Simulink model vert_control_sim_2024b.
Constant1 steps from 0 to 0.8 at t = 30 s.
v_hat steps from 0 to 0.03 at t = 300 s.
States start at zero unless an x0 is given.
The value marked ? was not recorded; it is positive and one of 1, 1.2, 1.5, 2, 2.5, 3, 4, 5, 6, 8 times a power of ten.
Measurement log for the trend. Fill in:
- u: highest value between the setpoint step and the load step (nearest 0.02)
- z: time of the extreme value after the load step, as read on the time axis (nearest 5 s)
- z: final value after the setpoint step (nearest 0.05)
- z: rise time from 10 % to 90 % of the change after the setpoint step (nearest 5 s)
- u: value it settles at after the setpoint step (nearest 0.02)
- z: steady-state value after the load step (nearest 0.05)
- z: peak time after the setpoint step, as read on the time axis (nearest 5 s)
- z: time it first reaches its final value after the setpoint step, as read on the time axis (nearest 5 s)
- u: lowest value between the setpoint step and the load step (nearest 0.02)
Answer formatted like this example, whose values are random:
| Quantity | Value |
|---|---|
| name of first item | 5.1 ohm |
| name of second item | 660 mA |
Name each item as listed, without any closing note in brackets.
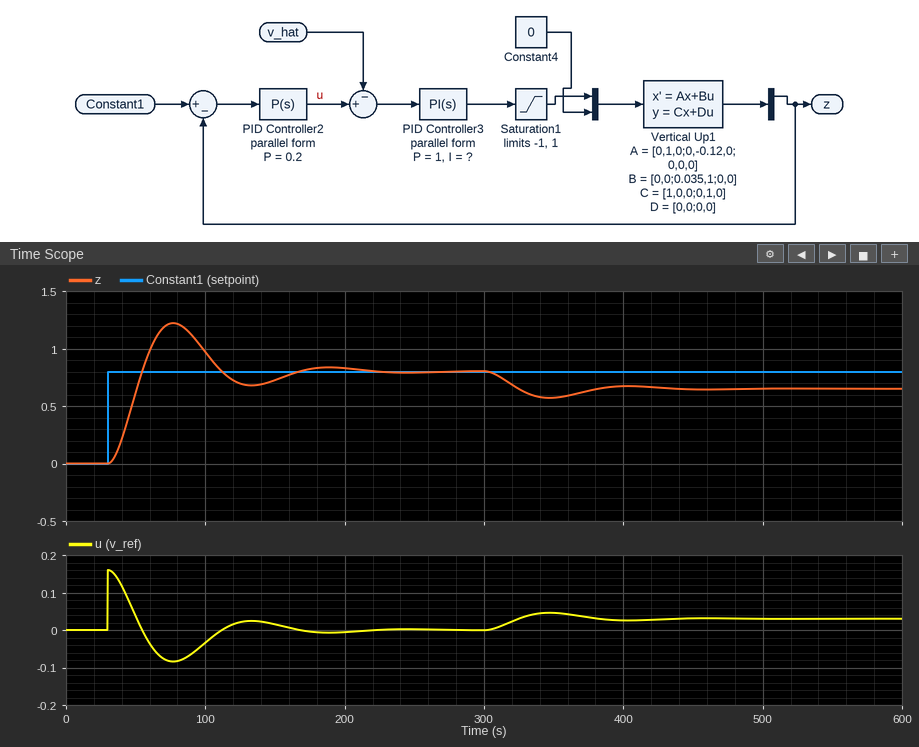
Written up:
| Quantity | Value |
|---|---|
| u: highest value between the setpoint step and the load step | 0.16 |
| z: time of the extreme value after the load step, as read on the time axis | 345 s |
| z: final value after the setpoint step | 0.80 |
| z: rise time from 10 % to 90 % of the change after the setpoint step | 15 s |
| u: value it settles at after the setpoint step | 0.00 |
| z: steady-state value after the load step | 0.65 |
| z: peak time after the setpoint step, as read on the time axis | 75 s |
| z: time it first reaches its final value after the setpoint step, as read on the time axis | 55 s |
| u: lowest value between the setpoint step and the load step | -0.08 |
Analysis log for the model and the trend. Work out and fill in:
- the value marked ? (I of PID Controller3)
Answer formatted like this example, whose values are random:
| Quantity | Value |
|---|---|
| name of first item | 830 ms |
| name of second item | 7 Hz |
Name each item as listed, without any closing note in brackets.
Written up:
| Quantity | Value |
|---|---|
| the value marked ? | 0.04 |
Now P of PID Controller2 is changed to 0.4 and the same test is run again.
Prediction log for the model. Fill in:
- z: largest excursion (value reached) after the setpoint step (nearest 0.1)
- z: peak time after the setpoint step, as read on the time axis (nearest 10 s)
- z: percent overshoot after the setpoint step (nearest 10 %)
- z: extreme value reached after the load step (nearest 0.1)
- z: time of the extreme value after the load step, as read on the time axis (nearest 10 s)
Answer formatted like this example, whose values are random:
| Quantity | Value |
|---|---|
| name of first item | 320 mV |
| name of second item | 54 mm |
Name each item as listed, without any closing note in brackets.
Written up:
| Quantity | Value |
|---|---|
| z: largest excursion (value reached) after the setpoint step | 1.2 |
| z: peak time after the setpoint step, as read on the time axis | 60 s |
| z: percent overshoot after the setpoint step | 50 % |
| z: extreme value reached after the load step | 0.7 |
| z: time of the extreme value after the load step, as read on the time axis | 330 s |
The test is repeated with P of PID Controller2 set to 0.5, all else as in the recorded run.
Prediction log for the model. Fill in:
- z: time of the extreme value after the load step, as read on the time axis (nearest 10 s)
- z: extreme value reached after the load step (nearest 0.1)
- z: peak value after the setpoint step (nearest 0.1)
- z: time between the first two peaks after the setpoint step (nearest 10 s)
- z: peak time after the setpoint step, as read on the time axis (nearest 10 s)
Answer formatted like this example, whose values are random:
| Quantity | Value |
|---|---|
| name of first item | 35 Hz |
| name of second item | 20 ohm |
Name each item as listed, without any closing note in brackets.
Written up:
| Quantity | Value |
|---|---|
| z: time of the extreme value after the load step, as read on the time axis | 330 s |
| z: extreme value reached after the load step | 0.7 |
| z: peak value after the setpoint step | 1.2 |
| z: time between the first two peaks after the setpoint step | 60 s |
| z: peak time after the setpoint step, as read on the time axis | 60 s |
